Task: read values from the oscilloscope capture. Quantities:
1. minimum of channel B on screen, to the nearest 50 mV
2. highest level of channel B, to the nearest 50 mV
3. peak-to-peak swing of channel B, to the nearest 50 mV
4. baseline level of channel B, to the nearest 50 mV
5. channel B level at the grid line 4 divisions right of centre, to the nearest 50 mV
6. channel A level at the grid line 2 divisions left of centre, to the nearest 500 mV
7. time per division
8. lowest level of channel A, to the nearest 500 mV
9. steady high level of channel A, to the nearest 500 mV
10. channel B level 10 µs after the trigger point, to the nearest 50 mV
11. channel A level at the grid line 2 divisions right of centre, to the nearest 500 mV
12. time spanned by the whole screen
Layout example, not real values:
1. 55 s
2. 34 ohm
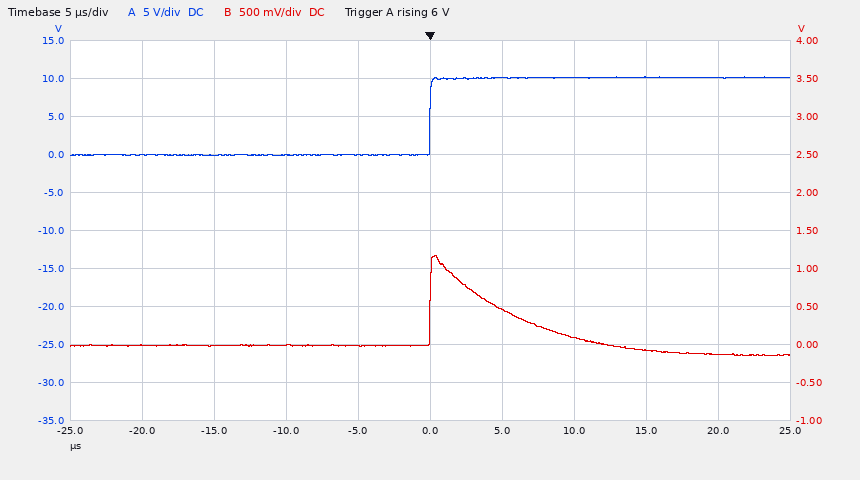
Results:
1. -150 mV
2. 1.15 V
3. 1.30 V
4. 0 mV
5. -150 mV
6. 0.0 V
7. 5 µs
8. 0.0 V
9. 10.0 V
10. 100 mV
11. 10.0 V
12. 50 µs
